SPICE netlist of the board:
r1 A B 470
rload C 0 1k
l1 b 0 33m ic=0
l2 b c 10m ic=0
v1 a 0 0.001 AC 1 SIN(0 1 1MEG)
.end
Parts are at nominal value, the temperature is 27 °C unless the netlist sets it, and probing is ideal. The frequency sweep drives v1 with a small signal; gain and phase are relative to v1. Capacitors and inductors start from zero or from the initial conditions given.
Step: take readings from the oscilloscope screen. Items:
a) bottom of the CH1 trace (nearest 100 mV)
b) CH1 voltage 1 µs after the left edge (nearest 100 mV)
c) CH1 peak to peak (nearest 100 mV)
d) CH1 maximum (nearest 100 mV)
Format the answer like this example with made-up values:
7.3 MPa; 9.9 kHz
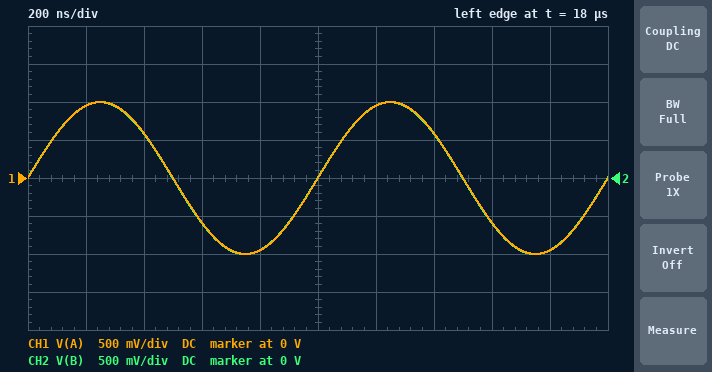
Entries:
-1.0 V; 0 V; 2.0 V; 1.0 V
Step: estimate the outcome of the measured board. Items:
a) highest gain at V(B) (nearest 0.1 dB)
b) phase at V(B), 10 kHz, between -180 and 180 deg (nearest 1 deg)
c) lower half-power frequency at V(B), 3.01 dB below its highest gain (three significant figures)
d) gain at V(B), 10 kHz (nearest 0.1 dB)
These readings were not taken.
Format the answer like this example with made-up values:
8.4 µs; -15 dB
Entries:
0 dB; 18 deg; 9.68 kHz; -3.0 dB
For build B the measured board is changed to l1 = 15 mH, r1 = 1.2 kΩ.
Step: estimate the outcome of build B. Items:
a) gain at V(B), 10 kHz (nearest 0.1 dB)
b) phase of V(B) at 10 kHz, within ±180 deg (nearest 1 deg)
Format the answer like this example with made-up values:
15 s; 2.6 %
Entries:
-8.3 dB; 44 deg
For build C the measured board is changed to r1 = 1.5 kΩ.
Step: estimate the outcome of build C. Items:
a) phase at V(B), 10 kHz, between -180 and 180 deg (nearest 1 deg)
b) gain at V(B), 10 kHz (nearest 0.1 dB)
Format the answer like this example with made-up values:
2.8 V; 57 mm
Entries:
34 deg; -8.0 dB
